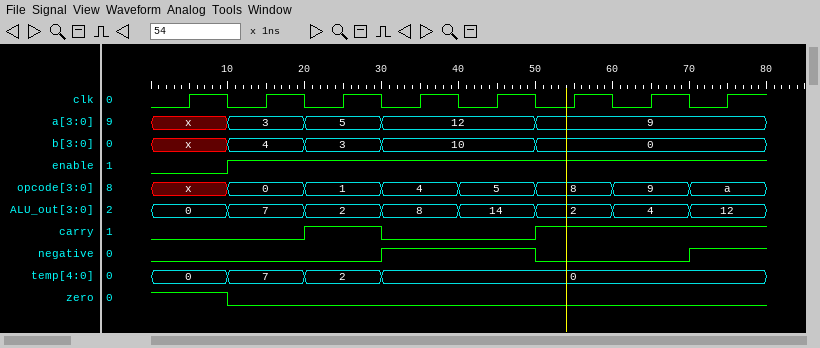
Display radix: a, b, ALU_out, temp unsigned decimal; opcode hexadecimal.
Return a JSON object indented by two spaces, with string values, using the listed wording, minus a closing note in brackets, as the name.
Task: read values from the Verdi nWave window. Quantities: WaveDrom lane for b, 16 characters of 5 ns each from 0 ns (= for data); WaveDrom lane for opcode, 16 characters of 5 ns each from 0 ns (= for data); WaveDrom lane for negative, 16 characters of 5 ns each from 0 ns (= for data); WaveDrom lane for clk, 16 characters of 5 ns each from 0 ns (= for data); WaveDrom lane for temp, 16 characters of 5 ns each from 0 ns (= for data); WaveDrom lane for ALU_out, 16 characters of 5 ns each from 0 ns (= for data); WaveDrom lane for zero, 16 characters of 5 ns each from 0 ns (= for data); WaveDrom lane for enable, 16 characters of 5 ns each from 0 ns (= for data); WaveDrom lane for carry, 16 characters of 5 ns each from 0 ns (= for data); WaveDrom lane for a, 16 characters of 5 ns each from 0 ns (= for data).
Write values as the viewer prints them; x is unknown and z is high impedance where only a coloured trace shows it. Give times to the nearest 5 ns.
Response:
{
  "WaveDrom lane for b, 16 characters of 5 ns each from 0 ns": "{name: 'b', wave: 'x.=.=.=...=.....', data: '4 3 10 0'}",
  "WaveDrom lane for opcode, 16 characters of 5 ns each from 0 ns": "{name: 'opcode', wave: 'x.=.=.=.=.=.=.=.', data: '0 1 4 5 8 9 a'}",
  "WaveDrom lane for negative, 16 characters of 5 ns each from 0 ns": "{name: 'negative', wave: '0.....1...0...1.'}",
  "WaveDrom lane for clk, 16 characters of 5 ns each from 0 ns": "{name: 'clk', wave: '0101010101010101'}",
  "WaveDrom lane for temp, 16 characters of 5 ns each from 0 ns": "{name: 'temp', wave: '=.=.=.=.........', data: '0 7 2 0'}",
  "WaveDrom lane for ALU_out, 16 characters of 5 ns each from 0 ns": "{name: 'ALU_out', wave: '=.=.=.=.=.=.=.=.', data: '0 7 2 8 14 2 4 12'}",
  "WaveDrom lane for zero, 16 characters of 5 ns each from 0 ns": "{name: 'zero', wave: '1.0.............'}",
  "WaveDrom lane for enable, 16 characters of 5 ns each from 0 ns": "{name: 'enable', wave: '0.1.............'}",
  "WaveDrom lane for carry, 16 characters of 5 ns each from 0 ns": "{name: 'carry', wave: '0...1.0...1.....'}",
  "WaveDrom lane for a, 16 characters of 5 ns each from 0 ns": "{name: 'a', wave: 'x.=.=.=...=.....', data: '3 5 12 9'}"
}
